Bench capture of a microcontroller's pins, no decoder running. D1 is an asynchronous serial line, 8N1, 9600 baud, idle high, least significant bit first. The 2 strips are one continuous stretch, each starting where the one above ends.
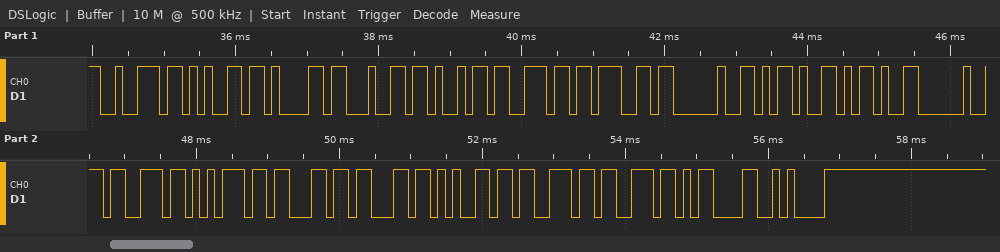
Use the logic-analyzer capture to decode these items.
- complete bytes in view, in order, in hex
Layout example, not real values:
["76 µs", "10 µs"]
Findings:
["72 65 61 64 69 6E 67 20 2D 2D 20 73 75 63 63 65 73 73 0D 0A"]
